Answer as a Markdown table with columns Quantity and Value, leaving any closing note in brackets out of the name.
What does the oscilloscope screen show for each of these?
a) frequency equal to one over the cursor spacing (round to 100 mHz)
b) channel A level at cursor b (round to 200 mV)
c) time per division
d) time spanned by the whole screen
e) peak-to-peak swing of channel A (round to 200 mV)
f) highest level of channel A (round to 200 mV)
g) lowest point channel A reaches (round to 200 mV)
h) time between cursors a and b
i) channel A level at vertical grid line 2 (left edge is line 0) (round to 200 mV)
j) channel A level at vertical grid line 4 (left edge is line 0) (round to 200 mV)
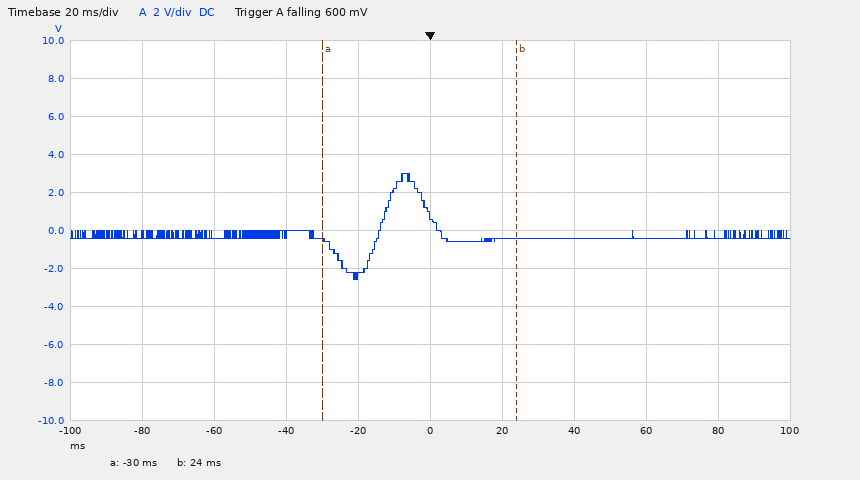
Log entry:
| Quantity | Value |
|---|---|
| frequency equal to one over the cursor spacing | 18.5 Hz |
| channel A level at cursor b | -400 mV |
| time per division | 20 ms |
| time spanned by the whole screen | 200 ms |
| peak-to-peak swing of channel A | 5.6 V |
| highest level of channel A | 3.0 V |
| lowest point channel A reaches | -2.6 V |
| time between cursors a and b | 54 ms |
| channel A level at vertical grid line 2 (left edge is line 0) | -200 mV |
| channel A level at vertical grid line 4 (left edge is line 0) | -2.4 V |
